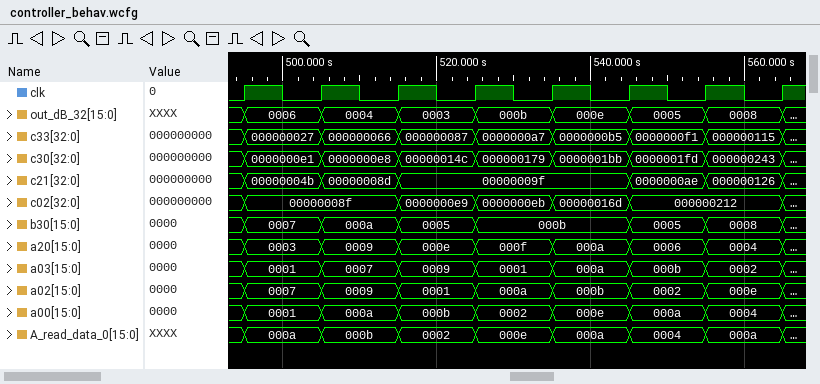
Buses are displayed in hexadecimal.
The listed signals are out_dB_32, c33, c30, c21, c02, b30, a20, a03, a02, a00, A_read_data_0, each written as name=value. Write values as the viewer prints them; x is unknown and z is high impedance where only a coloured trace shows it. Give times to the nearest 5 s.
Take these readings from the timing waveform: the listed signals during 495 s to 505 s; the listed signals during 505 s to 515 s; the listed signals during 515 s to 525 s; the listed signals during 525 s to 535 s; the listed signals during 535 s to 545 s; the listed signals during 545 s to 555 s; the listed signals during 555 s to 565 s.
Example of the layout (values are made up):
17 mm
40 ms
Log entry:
out_dB_32=0006, c33=000000027, c30=0000000e1, c21=00000004b, c02=00000008f, b30=0007, a20=0003, a03=0001, a02=0007, a00=0001, A_read_data_0=000a
out_dB_32=0004, c33=000000066, c30=0000000e8, c21=00000008d, c02=00000008f, b30=000a, a20=0009, a03=0007, a02=0009, a00=000a, A_read_data_0=000b
out_dB_32=0003, c33=000000087, c30=00000014c, c21=00000009f, c02=0000000e9, b30=0005, a20=000e, a03=0009, a02=0001, a00=000b, A_read_data_0=0002
out_dB_32=000b, c33=0000000a7, c30=000000179, c21=00000009f, c02=0000000eb, b30=000b, a20=000f, a03=0001, a02=000a, a00=0002, A_read_data_0=000e
out_dB_32=000e, c33=0000000b5, c30=0000001bb, c21=00000009f, c02=00000016d, b30=000b, a20=000a, a03=000a, a02=000b, a00=000e, A_read_data_0=000a
out_dB_32=0005, c33=0000000f1, c30=0000001fd, c21=0000000ae, c02=000000212, b30=0005, a20=0006, a03=000b, a02=0002, a00=000a, A_read_data_0=0004
out_dB_32=0008, c33=000000115, c30=000000243, c21=000000126, c02=000000212, b30=0008, a20=0004, a03=0002, a02=000e, a00=0004, A_read_data_0=000a
